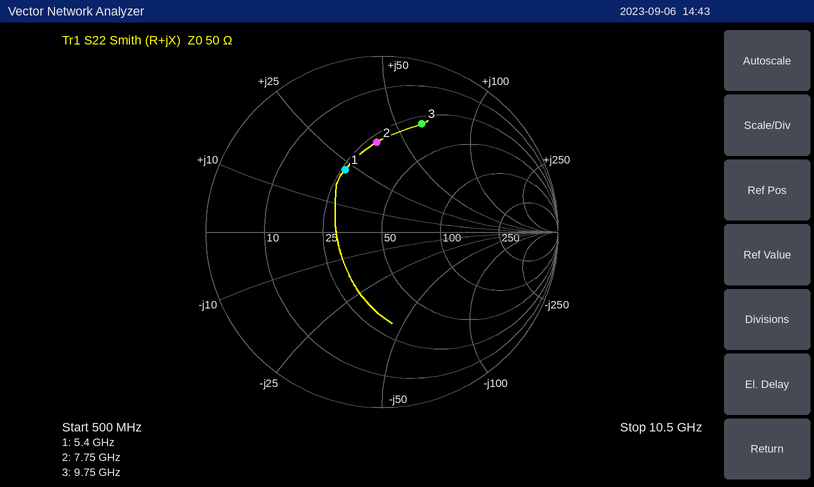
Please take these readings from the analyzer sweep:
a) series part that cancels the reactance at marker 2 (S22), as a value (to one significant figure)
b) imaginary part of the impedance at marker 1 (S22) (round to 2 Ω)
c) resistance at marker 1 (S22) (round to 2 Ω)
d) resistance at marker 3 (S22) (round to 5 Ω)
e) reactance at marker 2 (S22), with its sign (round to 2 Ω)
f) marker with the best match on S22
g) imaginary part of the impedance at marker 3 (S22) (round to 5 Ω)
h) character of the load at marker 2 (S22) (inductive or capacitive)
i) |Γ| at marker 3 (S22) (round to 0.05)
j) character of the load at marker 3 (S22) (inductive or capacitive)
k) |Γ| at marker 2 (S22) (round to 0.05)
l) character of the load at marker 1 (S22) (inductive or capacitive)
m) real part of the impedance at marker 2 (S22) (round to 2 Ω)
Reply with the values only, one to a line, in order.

500 fF
+22 Ω
26 Ω
30 Ω
+38 Ω
marker 1
+65 Ω
inductive
0.65
inductive
0.50
inductive
28 Ω
